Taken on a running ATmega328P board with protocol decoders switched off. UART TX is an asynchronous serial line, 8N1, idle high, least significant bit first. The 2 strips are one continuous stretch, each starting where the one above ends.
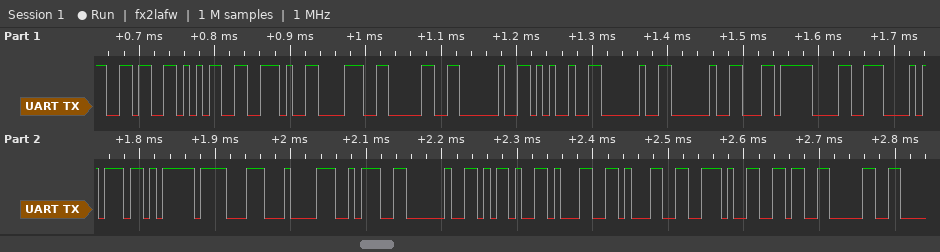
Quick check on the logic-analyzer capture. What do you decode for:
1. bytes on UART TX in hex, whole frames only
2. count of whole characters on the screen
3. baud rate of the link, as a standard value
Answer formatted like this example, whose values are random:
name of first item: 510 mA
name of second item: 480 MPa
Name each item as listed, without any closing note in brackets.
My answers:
bytes on UART TX in hex, whole frames only: 36 35 2E 38 30 20 25 20 20 EC 98 A8 EB 8F 84 3A 20 2D 31 31 2E 36 30
count of whole characters on the screen: 23
baud rate of the link, as a standard value: 115200 baud
